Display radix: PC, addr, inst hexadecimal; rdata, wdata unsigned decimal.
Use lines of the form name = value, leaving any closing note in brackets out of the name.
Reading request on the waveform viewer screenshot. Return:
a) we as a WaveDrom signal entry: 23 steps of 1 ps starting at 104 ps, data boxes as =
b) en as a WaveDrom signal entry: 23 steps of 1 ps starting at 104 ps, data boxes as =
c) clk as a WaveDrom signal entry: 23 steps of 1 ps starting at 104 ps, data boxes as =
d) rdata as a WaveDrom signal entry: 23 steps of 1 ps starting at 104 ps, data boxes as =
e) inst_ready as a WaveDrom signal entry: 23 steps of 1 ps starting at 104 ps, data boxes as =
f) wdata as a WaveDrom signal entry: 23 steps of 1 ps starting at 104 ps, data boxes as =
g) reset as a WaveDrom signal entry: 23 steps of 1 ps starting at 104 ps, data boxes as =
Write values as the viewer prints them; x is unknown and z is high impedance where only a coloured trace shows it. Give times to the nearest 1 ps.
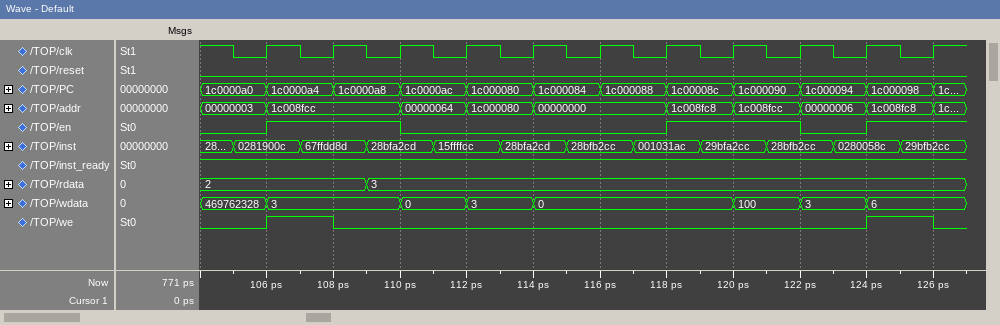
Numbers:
we as a WaveDrom signal entry: 23 steps of 1 ps starting at 104 ps, data boxes as = = {name: 'we', wave: '0.1.0...............1.0'}
en as a WaveDrom signal entry: 23 steps of 1 ps starting at 104 ps, data boxes as = = {name: 'en', wave: '0.1...0.......1...0.1..'}
clk as a WaveDrom signal entry: 23 steps of 1 ps starting at 104 ps, data boxes as = = {name: 'clk', wave: '10101010101010101010101'}
rdata as a WaveDrom signal entry: 23 steps of 1 ps starting at 104 ps, data boxes as = = {name: 'rdata', wave: '=....=.................', data: '2 3'}
inst_ready as a WaveDrom signal entry: 23 steps of 1 ps starting at 104 ps, data boxes as = = {name: 'inst_ready', wave: '1......................'}
wdata as a WaveDrom signal entry: 23 steps of 1 ps starting at 104 ps, data boxes as = = {name: 'wdata', wave: '=.=...=.=.=.....=.=.=..', data: '469762328 3 0 3 0 100 3 6'}
reset as a WaveDrom signal entry: 23 steps of 1 ps starting at 104 ps, data boxes as = = {name: 'reset', wave: '0......................'}
